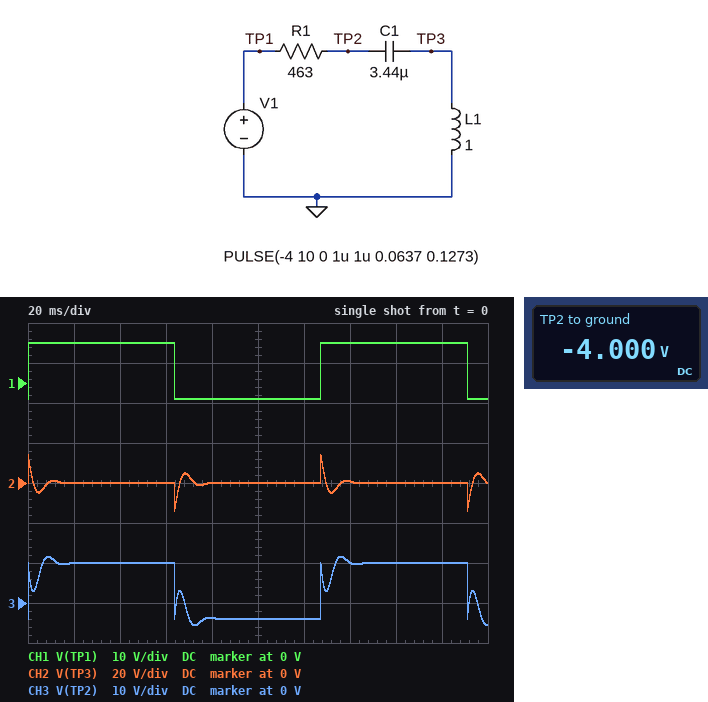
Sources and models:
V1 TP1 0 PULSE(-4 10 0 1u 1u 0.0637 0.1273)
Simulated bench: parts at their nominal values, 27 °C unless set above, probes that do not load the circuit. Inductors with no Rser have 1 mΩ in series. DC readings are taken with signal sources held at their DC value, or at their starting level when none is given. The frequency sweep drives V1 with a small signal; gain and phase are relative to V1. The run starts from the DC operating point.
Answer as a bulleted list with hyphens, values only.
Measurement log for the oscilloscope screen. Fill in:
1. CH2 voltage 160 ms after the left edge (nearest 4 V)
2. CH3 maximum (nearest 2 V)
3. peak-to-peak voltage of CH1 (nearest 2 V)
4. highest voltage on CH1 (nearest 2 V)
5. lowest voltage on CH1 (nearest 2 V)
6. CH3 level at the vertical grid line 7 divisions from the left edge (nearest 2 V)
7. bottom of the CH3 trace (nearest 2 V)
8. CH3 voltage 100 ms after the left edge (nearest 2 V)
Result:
- 0 V
- 12 V
- 14 V
- 10 V
- -4 V
- 10 V
- -6 V
- -4 V
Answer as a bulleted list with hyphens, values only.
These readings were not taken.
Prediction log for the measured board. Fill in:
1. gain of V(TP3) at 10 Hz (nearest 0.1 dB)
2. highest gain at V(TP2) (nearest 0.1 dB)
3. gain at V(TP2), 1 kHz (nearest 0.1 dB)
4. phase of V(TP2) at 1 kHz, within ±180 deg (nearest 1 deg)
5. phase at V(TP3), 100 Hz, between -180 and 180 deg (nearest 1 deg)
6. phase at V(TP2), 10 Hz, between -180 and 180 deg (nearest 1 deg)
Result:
- -37.3 dB
- 0 dB
- 0 dB
- 4 deg
- 70 deg
- -6 deg
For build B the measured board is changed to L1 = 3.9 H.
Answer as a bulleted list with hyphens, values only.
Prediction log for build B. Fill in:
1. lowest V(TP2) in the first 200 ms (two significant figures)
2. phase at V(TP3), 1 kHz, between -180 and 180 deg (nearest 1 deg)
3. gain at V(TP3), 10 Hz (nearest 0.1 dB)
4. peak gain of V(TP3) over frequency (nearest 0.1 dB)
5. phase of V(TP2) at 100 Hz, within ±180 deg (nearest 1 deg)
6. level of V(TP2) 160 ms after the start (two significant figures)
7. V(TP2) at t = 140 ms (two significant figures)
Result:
- -6.3 V
- 1 deg
- -25.1 dB
- 7.4 dB
- 13 deg
- 9.4 V
- 11 V
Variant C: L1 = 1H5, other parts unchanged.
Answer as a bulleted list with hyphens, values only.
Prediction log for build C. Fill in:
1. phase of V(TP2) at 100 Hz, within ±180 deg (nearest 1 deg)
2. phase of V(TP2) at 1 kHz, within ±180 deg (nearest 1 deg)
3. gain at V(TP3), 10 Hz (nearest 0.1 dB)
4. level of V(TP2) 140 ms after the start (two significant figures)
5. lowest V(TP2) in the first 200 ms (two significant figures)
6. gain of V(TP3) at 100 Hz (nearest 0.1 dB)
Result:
- 44 deg
- 3 deg
- -33.7 dB
- 11 V
- -5.9 V
- 3.0 dB
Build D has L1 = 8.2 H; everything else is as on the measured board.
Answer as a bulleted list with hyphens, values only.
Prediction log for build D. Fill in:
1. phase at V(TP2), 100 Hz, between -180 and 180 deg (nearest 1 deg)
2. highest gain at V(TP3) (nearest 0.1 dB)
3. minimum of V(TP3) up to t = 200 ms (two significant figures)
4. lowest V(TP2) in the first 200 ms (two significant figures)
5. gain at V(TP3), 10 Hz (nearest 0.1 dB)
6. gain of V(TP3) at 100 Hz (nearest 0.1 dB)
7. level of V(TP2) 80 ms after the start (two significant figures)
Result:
- 6 deg
- 10.6 dB
- -12 V
- -5.9 V
- -18.1 dB
- 0.8 dB
- -4.0 V
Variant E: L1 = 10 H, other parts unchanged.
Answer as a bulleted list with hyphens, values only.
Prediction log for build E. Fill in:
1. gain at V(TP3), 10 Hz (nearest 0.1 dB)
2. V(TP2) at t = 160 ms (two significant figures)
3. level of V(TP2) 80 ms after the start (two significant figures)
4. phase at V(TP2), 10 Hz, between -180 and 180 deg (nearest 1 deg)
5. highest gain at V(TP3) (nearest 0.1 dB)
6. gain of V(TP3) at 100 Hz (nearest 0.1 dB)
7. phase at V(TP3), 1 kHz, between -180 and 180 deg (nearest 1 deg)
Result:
- -16.1 dB
- 11 V
- -3.5 V
- -7 deg
- 11.4 dB
- 0.6 dB
- 0 deg
